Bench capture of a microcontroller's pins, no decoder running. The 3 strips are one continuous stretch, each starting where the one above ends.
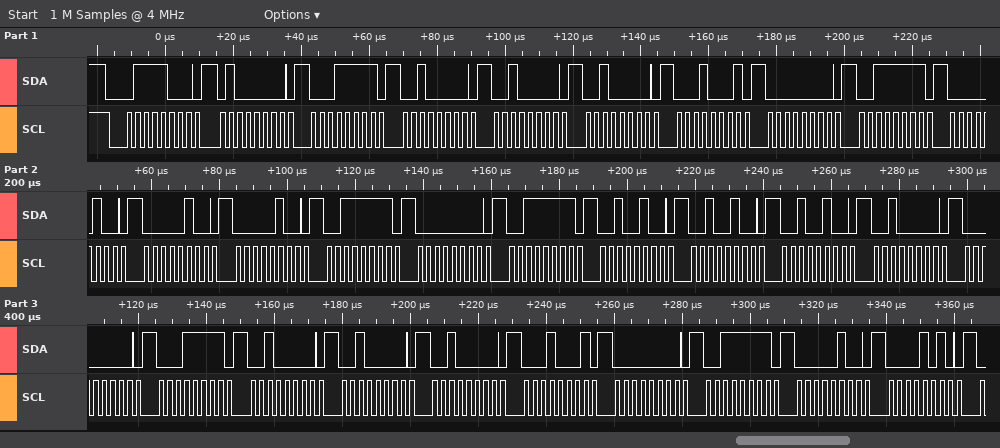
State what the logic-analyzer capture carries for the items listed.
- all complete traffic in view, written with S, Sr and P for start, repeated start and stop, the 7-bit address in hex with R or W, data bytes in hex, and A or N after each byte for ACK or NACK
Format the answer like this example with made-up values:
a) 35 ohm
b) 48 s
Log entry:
a) S 3CW A 40 A 1F A 20 A 20 A 20 A 11 A 00 A 3F A 04 A 04 A 04 A 3F A 00 A 3F A 24 A 24 A 24 A 20 A 00 A 1F A 20 A 20 A 20 A 11 A 00 A 3F A 04 A 0A A
